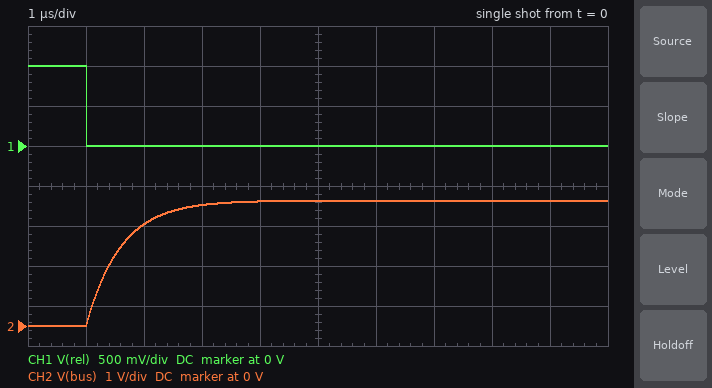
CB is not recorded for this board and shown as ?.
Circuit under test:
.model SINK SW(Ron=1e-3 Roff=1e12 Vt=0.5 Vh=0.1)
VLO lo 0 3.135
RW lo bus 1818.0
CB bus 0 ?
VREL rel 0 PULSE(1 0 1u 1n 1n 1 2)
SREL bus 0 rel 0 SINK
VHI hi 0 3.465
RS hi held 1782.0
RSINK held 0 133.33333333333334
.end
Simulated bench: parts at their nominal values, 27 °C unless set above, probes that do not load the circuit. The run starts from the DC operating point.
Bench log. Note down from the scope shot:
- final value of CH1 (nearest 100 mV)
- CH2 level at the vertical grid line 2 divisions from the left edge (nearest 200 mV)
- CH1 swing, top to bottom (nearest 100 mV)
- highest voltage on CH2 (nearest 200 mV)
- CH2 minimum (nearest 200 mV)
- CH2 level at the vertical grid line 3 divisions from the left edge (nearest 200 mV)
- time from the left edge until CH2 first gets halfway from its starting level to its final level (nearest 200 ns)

0 V
2.6 V
1.0 V
3.2 V
0 V
3.0 V
1.4 µs
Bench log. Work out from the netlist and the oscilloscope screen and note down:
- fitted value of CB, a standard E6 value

330 pF
